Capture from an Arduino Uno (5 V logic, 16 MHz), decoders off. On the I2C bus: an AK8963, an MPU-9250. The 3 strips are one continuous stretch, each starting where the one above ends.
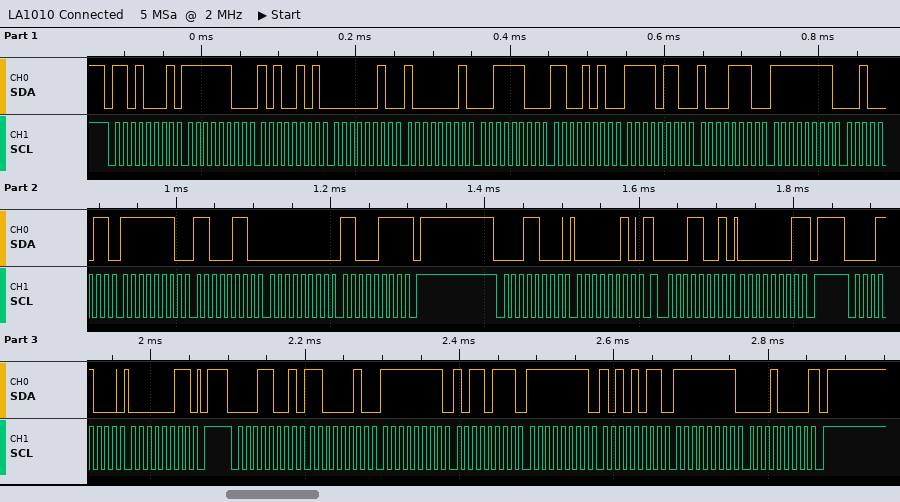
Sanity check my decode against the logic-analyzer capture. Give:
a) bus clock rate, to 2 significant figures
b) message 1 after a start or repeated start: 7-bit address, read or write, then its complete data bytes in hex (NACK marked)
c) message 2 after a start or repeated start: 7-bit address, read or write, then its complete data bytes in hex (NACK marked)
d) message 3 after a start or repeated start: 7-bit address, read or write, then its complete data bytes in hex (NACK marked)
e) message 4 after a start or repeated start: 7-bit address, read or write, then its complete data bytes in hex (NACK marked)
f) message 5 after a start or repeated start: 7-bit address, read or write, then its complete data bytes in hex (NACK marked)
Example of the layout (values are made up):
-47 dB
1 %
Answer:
100 kHz
0x68 read: FC A5 02 81 3C CA F6 8E FF 23 FE C6 00 C7 NACK
0x0C write: 02
0x0C read: 01 NACK
0x0C write: 03
0x0C read: C2 FF B7 FF AB FF 10 NACK
